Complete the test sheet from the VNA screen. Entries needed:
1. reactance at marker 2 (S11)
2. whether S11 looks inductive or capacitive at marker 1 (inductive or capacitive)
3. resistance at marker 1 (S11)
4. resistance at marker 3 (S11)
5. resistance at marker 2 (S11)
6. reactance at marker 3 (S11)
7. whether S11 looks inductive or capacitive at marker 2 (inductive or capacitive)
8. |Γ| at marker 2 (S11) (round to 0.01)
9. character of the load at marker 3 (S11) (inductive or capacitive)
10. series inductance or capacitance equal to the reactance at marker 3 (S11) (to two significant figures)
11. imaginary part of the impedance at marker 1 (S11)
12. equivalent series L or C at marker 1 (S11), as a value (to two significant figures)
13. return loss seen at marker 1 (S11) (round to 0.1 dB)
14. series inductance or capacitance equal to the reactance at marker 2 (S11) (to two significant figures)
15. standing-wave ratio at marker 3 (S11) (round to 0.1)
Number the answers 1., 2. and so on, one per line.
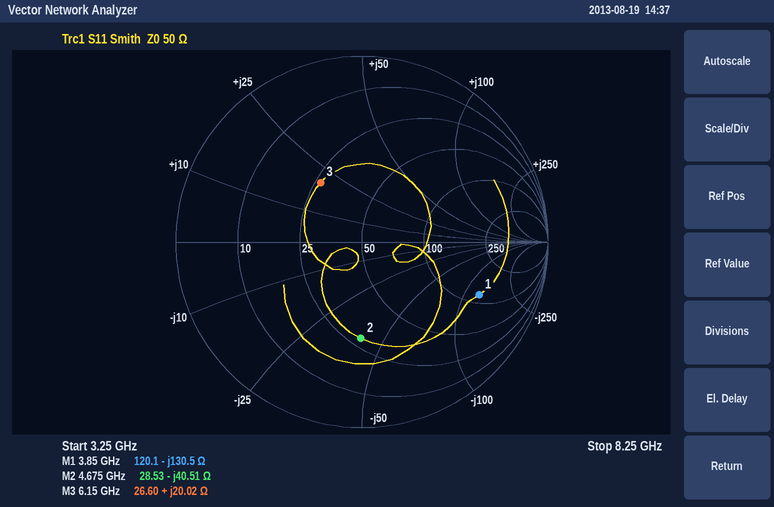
1. -40.51 Ω
2. capacitive
3. 120.1 Ω
4. 26.60 Ω
5. 28.53 Ω
6. +20.02 Ω
7. capacitive
8. 0.52
9. inductive
10. 520 pH
11. -130.5 Ω
12. 320 fF
13. 3.2 dB
14. 840 fF
15. 2.3
